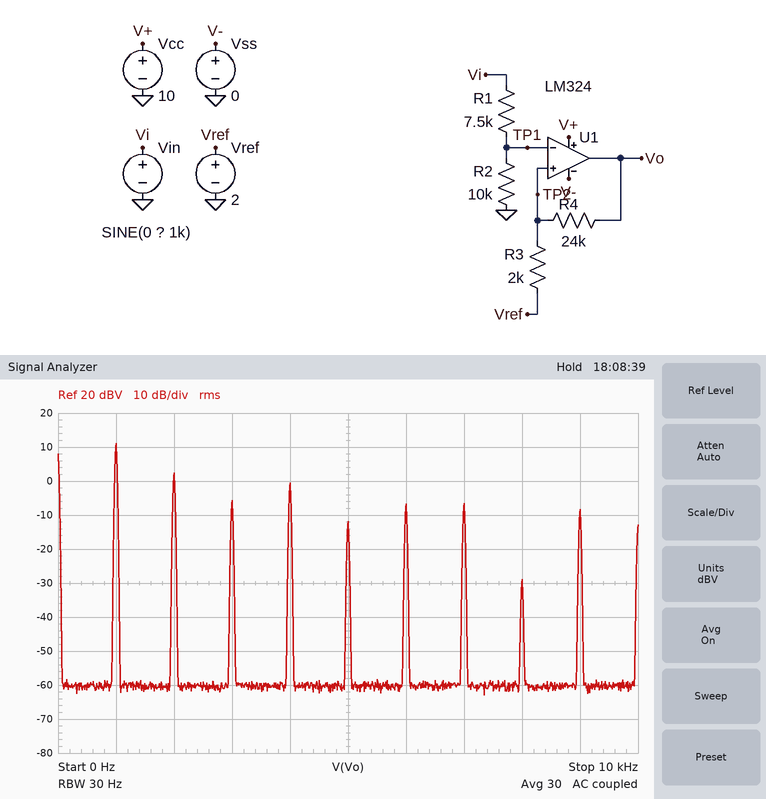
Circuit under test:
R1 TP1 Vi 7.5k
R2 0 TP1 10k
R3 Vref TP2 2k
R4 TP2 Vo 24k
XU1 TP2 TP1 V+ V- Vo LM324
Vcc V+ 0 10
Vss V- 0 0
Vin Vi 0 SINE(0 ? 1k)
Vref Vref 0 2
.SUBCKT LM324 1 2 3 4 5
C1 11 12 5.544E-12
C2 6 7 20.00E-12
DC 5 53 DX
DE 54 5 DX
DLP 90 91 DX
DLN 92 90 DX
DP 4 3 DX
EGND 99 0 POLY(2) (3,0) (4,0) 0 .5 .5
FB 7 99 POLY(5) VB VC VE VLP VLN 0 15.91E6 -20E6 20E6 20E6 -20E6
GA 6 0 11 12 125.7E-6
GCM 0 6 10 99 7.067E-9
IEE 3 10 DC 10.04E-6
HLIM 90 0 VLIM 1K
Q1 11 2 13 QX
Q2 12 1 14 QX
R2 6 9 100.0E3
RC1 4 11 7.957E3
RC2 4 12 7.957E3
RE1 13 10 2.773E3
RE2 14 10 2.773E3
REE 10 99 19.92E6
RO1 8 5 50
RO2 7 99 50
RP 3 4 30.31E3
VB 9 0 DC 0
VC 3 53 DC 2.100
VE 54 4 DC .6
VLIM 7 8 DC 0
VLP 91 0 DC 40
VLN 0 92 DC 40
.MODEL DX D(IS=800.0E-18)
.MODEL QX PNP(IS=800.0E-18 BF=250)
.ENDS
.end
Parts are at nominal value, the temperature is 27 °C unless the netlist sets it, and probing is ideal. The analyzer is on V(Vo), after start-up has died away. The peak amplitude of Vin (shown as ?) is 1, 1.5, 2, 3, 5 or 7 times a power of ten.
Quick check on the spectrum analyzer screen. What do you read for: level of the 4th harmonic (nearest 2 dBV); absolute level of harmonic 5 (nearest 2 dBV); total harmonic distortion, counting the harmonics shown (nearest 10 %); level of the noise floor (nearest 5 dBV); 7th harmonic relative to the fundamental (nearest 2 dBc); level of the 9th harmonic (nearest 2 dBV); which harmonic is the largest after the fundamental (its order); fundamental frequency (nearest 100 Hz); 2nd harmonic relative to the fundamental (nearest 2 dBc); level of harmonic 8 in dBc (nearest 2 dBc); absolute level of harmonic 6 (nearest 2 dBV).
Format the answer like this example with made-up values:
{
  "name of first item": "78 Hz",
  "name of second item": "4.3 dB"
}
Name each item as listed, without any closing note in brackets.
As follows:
{
  "level of the 4th harmonic": "0 dBV",
  "absolute level of harmonic 5": "-12 dBV",
  "total harmonic distortion, counting the harmonics shown": "50 %",
  "level of the noise floor": "-60 dBV",
  "7th harmonic relative to the fundamental": "-18 dBc",
  "level of the 9th harmonic": "-8 dBV",
  "which harmonic is the largest after the fundamental": "2",
  "fundamental frequency": "1.0 kHz",
  "2nd harmonic relative to the fundamental": "-8 dBc",
  "level of harmonic 8 in dBc": "-40 dBc",
  "absolute level of harmonic 6": "-6 dBV"
}
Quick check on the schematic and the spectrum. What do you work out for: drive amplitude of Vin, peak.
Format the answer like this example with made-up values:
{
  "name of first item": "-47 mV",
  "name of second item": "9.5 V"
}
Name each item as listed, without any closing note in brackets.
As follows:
{
  "drive amplitude of Vin, peak": "3 V"
}
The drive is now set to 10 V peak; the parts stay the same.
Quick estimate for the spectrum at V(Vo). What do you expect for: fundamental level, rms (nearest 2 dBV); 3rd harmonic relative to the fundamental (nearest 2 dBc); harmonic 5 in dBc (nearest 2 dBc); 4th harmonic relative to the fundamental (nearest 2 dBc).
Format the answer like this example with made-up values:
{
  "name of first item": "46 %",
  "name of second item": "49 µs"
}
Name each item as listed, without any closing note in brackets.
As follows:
{
  "fundamental level, rms": "-8 dBV",
  "3rd harmonic relative to the fundamental": "6 dBc",
  "harmonic 5 in dBc": "8 dBc",
  "4th harmonic relative to the fundamental": "10 dBc"
}
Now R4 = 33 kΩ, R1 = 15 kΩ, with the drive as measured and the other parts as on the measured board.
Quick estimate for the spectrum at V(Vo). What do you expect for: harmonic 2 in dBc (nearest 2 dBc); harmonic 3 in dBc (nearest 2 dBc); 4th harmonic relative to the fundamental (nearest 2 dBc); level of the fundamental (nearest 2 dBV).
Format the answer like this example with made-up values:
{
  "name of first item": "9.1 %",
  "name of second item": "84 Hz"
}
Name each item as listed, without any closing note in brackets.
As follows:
{
  "harmonic 2 in dBc": "-6 dBc",
  "harmonic 3 in dBc": "-22 dBc",
  "4th harmonic relative to the fundamental": "-14 dBc",
  "level of the fundamental": "10 dBV"
}
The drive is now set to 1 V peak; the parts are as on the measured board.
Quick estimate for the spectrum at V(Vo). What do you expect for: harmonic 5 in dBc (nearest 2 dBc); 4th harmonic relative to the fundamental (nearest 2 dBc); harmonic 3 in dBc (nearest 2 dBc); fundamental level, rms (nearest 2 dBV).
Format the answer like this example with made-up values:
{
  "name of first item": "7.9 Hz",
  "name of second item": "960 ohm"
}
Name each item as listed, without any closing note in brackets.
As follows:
{
  "harmonic 5 in dBc": "-10 dBc",
  "4th harmonic relative to the fundamental": "-6 dBc",
  "harmonic 3 in dBc": "-2 dBc",
  "fundamental level, rms": "-50 dBV"
}
